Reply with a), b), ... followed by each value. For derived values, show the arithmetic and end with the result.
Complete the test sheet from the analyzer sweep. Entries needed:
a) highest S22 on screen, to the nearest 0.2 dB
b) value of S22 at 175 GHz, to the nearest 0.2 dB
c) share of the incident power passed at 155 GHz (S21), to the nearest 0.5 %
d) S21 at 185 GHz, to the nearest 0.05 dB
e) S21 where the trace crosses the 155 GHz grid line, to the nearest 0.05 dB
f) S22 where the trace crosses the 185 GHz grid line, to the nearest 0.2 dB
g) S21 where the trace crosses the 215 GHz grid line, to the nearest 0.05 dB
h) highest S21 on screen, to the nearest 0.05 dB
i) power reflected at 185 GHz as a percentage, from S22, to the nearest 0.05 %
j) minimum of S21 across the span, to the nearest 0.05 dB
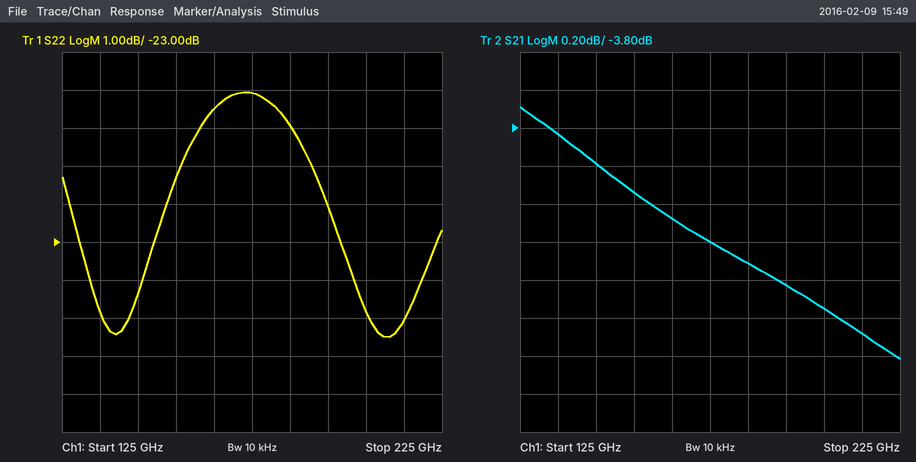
a) -19.0 dB
b) -19.0 dB
c) 10^(-4.15/10) ≈ 38.5 %
d) -4.50 dB
e) -4.15 dB
f) -20.0 dB
g) -4.90 dB
h) -3.70 dB
i) 10^(-20/10) ≈ 1.00 %
j) -5.00 dB
